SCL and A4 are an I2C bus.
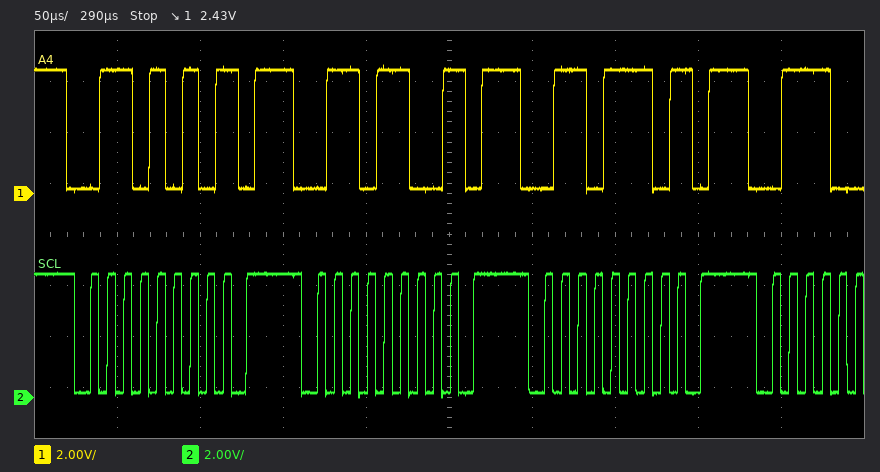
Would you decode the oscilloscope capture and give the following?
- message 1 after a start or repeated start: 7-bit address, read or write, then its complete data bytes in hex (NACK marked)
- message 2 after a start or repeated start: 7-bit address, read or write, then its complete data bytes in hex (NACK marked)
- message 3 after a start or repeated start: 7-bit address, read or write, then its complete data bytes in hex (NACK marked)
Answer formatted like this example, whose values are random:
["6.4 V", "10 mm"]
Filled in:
["0x35 write NACK", "0x36 write NACK", "0x37 write NACK"]
